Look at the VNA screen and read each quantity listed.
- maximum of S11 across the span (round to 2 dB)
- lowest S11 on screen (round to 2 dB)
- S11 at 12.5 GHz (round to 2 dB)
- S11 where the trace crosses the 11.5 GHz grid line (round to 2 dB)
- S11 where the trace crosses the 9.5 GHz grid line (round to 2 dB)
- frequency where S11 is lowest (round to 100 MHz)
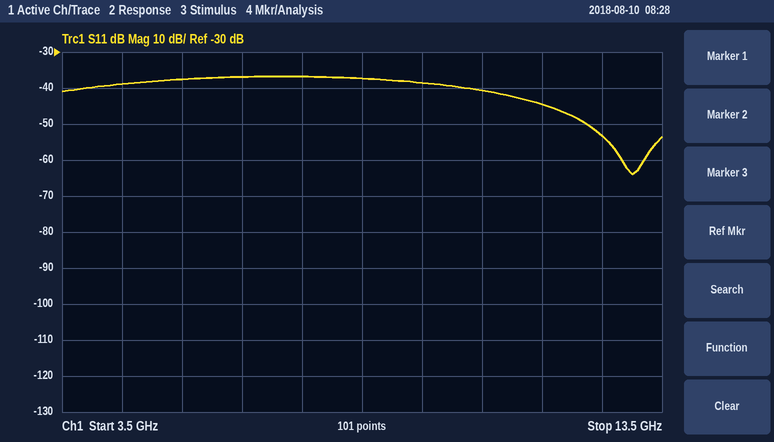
-36 dB
-64 dB
-54 dB
-44 dB
-38 dB
13.0 GHz
